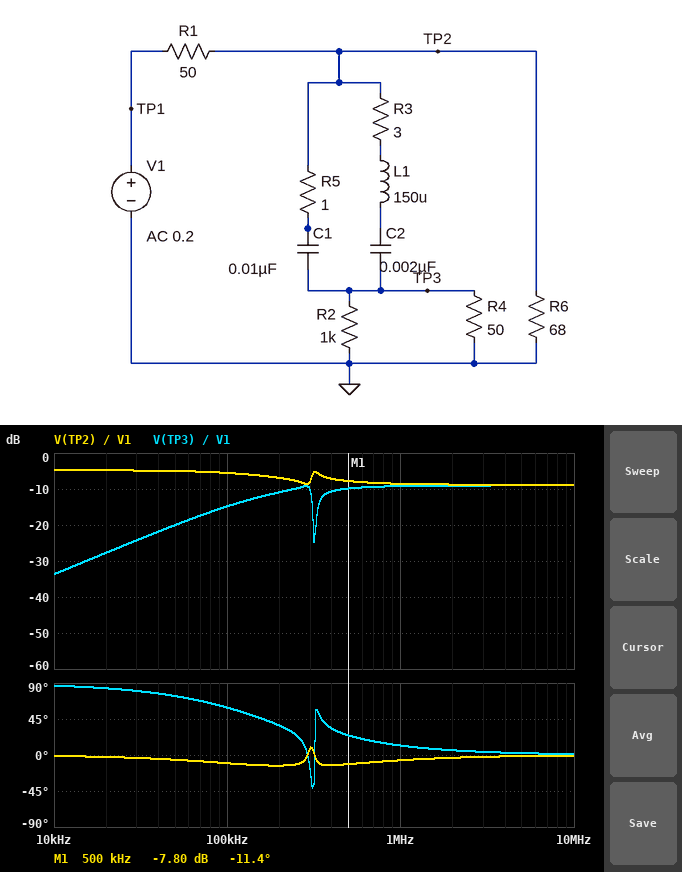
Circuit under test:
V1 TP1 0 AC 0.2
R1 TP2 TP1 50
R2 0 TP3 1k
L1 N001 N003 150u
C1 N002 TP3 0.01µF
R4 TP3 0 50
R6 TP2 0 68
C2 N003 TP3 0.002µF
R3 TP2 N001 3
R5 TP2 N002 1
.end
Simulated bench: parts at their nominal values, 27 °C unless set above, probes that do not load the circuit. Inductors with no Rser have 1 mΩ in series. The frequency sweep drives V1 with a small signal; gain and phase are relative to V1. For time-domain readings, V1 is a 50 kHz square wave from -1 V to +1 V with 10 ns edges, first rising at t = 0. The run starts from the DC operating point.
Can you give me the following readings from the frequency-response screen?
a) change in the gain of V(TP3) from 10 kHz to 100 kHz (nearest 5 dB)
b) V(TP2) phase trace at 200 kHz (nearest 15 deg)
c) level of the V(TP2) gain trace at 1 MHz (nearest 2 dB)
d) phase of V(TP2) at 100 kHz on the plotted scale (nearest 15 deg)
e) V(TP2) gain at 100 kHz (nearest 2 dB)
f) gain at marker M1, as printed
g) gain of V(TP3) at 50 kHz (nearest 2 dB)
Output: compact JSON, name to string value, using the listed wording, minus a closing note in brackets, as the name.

{"change in the gain of V(TP3) from 10 kHz to 100 kHz": "20 dB", "V(TP2) phase trace at 200 kHz": "-15 deg", "level of the V(TP2) gain trace at 1 MHz": "-8 dB", "phase of V(TP2) at 100 kHz on the plotted scale": "-15 deg", "V(TP2) gain at 100 kHz": "-6 dB", "gain at marker M1, as printed": "-7.80 dB", "gain of V(TP3) at 50 kHz": "-20 dB"}
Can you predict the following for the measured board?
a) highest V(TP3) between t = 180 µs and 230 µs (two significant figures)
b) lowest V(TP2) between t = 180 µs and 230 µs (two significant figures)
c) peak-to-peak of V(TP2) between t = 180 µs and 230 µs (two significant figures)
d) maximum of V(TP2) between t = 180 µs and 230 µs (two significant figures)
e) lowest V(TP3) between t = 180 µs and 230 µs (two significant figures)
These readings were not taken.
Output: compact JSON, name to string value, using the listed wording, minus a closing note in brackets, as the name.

{"highest V(TP3) between t = 180 µs and 230 µs": "720 mV", "lowest V(TP2) between t = 180 µs and 230 µs": "-590 mV", "peak-to-peak of V(TP2) between t = 180 µs and 230 µs": "1.2 V", "maximum of V(TP2) between t = 180 µs and 230 µs": "590 mV", "lowest V(TP3) between t = 180 µs and 230 µs": "-720 mV"}
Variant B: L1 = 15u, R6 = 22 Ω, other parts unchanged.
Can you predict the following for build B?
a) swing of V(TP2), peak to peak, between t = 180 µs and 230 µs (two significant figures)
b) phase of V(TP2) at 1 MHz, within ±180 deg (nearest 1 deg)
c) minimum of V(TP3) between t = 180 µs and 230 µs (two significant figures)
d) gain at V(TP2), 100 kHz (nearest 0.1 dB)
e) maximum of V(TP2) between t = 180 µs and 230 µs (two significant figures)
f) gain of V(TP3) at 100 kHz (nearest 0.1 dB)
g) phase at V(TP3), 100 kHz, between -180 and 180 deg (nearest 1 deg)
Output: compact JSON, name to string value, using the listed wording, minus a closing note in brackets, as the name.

{"swing of V(TP2), peak to peak, between t = 180 µs and 230 µs": "610 mV", "phase of V(TP2) at 1 MHz, within ±180 deg": "1 deg", "minimum of V(TP3) between t = 180 µs and 230 µs": "-450 mV", "gain at V(TP2), 100 kHz": "-10.7 dB", "maximum of V(TP2) between t = 180 µs and 230 µs": "310 mV", "gain of V(TP3) at 100 kHz": "-20.1 dB", "phase at V(TP3), 100 kHz, between -180 and 180 deg": "64 deg"}
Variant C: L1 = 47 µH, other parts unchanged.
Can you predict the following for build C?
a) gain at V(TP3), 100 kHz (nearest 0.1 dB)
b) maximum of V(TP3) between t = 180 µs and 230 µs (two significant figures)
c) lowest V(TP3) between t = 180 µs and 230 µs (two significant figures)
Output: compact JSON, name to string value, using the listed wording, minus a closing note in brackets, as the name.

{"gain at V(TP3), 100 kHz": "-14.9 dB", "maximum of V(TP3) between t = 180 µs and 230 µs": "690 mV", "lowest V(TP3) between t = 180 µs and 230 µs": "-690 mV"}
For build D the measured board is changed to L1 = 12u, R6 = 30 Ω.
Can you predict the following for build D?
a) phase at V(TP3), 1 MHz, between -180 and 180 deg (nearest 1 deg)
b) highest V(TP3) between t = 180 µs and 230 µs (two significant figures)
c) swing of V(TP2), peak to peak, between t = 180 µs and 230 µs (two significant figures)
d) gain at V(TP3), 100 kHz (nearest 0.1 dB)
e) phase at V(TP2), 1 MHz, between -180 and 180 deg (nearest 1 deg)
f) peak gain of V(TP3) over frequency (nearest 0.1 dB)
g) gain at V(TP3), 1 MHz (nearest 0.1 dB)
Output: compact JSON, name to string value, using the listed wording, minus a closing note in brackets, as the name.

{"phase at V(TP3), 1 MHz, between -180 and 180 deg": "3 deg", "highest V(TP3) between t = 180 µs and 230 µs": "530 mV", "swing of V(TP2), peak to peak, between t = 180 µs and 230 µs": "750 mV", "gain at V(TP3), 100 kHz": "-18.4 dB", "phase at V(TP2), 1 MHz, between -180 and 180 deg": "-1 deg", "peak gain of V(TP3) over frequency": "-11.5 dB", "gain at V(TP3), 1 MHz": "-11.7 dB"}
